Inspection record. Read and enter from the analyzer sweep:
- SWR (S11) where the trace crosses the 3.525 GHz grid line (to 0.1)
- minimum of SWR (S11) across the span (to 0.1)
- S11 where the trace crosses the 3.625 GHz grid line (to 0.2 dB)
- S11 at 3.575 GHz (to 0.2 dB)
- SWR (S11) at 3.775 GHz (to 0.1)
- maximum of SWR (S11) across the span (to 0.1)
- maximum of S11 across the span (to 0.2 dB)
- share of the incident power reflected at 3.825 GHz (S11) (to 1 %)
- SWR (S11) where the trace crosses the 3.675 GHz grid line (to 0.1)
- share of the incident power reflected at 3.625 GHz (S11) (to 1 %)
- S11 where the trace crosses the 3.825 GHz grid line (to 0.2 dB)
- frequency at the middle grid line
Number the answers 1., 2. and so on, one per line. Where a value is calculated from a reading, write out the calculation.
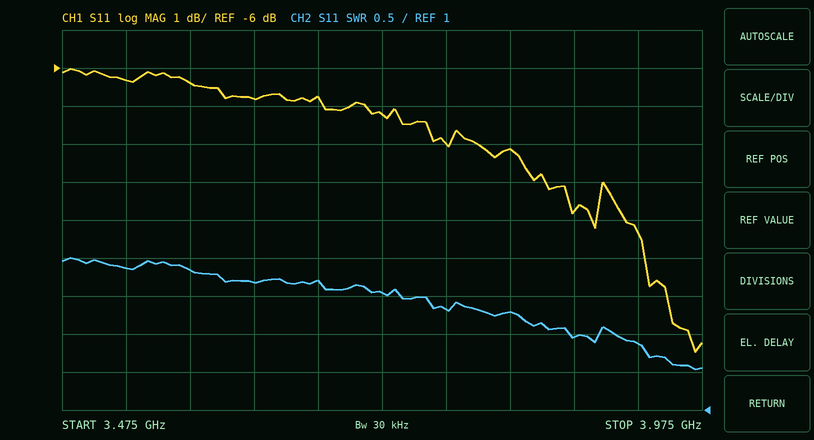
1. 2.9
2. 1.5
3. -6.8 dB
4. -6.4 dB
5. 2.3
6. 3.0
7. -6.0 dB
8. 10^(-8.2/10) ≈ 15 %
9. 2.7
10. 10^(-6.8/10) ≈ 21 %
11. -8.2 dB
12. 3.725 GHz
